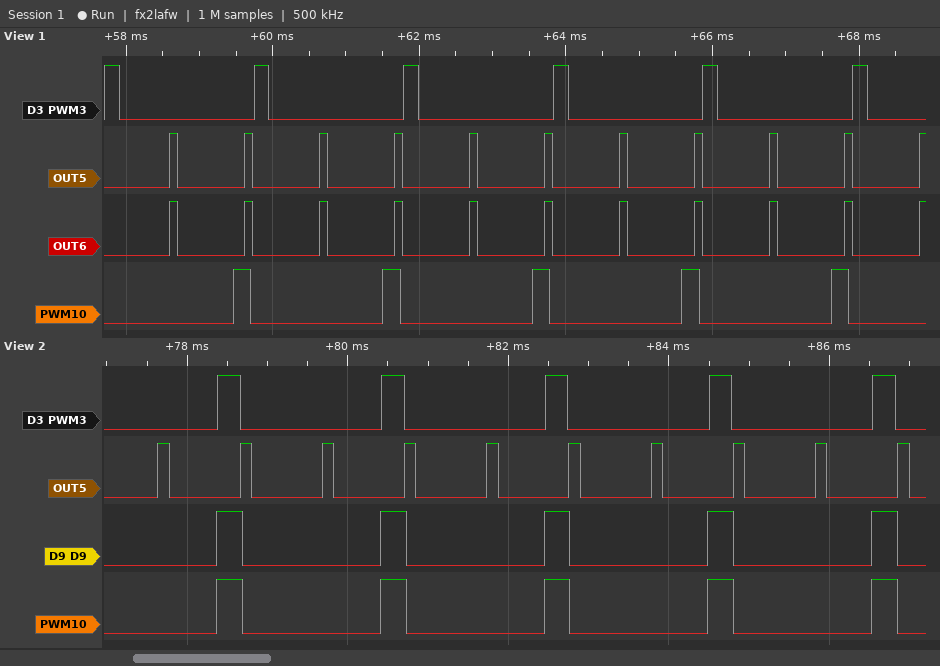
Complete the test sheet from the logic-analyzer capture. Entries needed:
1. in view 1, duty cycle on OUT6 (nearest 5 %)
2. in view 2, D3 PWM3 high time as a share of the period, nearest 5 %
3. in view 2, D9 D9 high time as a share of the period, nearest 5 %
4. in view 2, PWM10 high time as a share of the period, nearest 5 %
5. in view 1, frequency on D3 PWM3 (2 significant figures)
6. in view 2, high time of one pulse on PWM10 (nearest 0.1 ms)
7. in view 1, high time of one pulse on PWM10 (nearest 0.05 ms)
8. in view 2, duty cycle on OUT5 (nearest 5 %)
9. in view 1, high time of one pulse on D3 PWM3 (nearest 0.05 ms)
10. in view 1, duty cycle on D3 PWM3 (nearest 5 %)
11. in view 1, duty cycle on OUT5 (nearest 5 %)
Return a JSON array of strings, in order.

["10 %", "15 %", "15 %", "15 %", "490 Hz", "0.3 ms", "0.25 ms", "15 %", "0.20 ms", "10 %", "10 %"]
